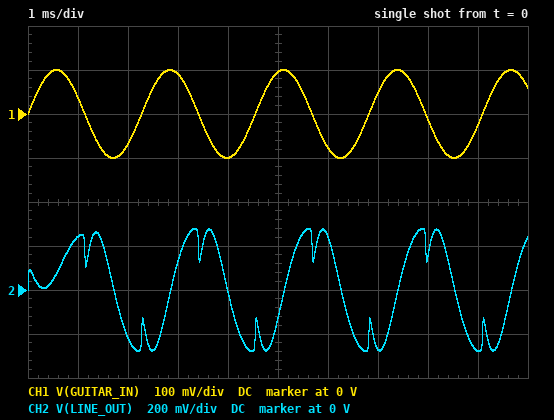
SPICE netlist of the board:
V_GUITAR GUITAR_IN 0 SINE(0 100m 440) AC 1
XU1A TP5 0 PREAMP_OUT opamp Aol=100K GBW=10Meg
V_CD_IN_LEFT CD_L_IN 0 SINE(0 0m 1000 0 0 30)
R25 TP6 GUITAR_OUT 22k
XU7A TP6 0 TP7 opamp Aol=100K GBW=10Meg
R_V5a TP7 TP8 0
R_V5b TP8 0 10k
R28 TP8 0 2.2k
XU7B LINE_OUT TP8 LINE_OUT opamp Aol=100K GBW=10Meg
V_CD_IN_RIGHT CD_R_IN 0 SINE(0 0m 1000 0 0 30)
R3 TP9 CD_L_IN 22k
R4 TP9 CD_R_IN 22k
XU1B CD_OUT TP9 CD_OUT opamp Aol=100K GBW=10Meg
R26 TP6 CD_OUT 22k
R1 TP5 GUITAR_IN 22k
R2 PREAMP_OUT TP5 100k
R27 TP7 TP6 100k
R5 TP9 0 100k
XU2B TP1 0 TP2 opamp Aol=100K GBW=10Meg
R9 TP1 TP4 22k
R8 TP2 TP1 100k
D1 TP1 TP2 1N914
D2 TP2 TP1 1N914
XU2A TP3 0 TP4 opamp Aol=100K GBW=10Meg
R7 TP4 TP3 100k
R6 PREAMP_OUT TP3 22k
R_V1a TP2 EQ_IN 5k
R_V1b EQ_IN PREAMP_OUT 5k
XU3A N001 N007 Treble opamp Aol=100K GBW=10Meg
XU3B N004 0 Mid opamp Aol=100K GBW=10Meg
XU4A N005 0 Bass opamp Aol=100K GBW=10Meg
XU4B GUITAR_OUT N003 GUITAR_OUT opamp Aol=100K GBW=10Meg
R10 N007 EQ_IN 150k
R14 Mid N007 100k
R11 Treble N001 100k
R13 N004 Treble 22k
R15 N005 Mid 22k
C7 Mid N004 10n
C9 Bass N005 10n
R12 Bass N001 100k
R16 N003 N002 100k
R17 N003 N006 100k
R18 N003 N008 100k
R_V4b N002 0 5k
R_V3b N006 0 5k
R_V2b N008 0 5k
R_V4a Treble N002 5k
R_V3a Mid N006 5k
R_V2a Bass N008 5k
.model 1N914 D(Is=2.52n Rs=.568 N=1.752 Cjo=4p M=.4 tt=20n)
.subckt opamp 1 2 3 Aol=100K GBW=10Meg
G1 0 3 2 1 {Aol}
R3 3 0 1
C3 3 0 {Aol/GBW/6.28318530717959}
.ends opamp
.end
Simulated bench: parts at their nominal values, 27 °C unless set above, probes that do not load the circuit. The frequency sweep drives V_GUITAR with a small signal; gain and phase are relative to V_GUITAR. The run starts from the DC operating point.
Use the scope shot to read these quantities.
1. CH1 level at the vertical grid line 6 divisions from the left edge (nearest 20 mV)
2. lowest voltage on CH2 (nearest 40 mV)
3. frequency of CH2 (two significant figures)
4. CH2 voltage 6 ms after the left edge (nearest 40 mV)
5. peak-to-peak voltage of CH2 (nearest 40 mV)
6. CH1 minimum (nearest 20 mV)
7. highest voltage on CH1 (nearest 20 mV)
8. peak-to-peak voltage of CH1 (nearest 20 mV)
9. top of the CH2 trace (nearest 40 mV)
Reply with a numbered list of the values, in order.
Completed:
1. -80 mV
2. -280 mV
3. 440 Hz
4. 240 mV
5. 560 mV
6. -100 mV
7. 100 mV
8. 200 mV
9. 280 mV
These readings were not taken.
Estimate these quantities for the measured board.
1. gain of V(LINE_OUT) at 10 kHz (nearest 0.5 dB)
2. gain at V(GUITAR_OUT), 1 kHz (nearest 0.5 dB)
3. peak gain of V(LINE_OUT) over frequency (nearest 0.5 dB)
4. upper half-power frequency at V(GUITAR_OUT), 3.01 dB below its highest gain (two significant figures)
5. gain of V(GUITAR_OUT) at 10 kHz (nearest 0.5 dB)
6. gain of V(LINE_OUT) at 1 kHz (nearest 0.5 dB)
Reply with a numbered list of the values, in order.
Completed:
1. 29.5 dB
2. 15.0 dB
3. 29.5 dB
4. 180 kHz
5. 16.0 dB
6. 28.0 dB
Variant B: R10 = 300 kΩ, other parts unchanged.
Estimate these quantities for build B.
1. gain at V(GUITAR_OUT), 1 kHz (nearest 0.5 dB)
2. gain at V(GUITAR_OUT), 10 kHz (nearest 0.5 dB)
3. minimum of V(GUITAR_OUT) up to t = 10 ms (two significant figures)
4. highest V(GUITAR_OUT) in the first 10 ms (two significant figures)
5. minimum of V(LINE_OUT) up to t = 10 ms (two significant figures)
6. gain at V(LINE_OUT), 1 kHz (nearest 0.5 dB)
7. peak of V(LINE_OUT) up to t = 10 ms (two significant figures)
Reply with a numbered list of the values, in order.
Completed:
1. 9.5 dB
2. 12.0 dB
3. -36 mV
4. 36 mV
5. -160 mV
6. 22.5 dB
7. 160 mV
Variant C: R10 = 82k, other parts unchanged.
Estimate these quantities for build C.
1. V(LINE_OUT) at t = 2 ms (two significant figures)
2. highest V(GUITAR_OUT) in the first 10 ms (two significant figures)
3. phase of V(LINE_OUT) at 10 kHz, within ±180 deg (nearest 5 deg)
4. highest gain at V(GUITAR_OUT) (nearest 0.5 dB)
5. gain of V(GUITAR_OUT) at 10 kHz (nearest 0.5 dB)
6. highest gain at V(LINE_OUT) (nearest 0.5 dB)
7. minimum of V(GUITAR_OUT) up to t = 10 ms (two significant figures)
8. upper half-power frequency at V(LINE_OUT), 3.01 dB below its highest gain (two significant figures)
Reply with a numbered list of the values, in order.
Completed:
1. -380 mV
2. 100 mV
3. 5 deg
4. 19.5 dB
5. 19.0 dB
6. 33.0 dB
7. -100 mV
8. 140 kHz
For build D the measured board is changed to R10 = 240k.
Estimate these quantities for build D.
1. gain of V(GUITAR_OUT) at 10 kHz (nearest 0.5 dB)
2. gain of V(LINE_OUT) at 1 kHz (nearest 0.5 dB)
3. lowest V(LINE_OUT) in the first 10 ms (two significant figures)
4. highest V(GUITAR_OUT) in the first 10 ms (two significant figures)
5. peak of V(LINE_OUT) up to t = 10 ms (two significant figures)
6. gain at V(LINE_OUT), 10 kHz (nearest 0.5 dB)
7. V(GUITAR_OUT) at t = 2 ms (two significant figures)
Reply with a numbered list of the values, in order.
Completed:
1. 13.5 dB
2. 24.5 dB
3. -200 mV
4. 43 mV
5. 200 mV
6. 26.5 dB
7. 30 mV
